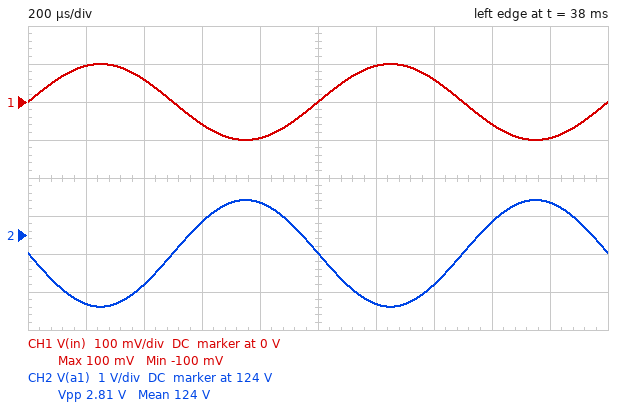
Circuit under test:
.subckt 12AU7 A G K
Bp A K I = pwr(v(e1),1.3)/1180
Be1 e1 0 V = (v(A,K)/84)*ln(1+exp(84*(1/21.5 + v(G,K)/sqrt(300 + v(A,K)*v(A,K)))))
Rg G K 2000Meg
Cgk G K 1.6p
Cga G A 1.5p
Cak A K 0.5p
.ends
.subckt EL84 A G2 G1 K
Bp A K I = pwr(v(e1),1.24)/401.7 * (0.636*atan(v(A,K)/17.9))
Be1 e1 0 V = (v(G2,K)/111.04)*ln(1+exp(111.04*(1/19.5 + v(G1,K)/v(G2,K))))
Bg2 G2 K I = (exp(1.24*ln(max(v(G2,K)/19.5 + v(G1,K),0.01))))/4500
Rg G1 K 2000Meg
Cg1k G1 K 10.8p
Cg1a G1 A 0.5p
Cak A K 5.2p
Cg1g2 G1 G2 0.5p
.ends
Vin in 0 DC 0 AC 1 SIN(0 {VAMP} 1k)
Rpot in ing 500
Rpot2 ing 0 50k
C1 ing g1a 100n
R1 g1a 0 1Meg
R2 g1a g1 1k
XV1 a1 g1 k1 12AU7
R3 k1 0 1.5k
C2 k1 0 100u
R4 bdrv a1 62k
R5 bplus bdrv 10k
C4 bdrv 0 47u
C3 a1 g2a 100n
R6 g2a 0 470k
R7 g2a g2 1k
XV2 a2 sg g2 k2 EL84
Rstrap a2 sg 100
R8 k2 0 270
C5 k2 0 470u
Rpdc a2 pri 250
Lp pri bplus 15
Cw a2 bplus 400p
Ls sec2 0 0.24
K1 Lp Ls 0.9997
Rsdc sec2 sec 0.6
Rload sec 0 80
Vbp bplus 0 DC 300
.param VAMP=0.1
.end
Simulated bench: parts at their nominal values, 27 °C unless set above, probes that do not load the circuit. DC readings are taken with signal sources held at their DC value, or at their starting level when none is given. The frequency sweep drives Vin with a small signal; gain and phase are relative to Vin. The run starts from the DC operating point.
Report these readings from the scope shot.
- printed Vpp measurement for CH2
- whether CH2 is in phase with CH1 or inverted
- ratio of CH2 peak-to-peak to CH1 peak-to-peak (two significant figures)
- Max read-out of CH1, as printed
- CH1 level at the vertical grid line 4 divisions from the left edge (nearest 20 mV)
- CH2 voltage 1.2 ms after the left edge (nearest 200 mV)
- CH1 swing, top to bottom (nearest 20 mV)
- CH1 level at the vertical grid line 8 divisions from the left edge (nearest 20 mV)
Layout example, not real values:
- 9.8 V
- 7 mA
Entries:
- 2.81 V
- inverted
- 14
- 100 mV
- -100 mV
- 122.2 V
- 200 mV
- -60 mV
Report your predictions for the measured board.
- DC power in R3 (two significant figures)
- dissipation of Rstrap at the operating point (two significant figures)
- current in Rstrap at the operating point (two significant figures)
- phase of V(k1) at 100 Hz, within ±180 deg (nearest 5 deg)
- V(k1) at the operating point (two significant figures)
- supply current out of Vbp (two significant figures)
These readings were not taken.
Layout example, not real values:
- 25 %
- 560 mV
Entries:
- 9.0 mW
- 570 µW
- 2.4 mA
- -90 deg
- 3.7 V
- 31 mA
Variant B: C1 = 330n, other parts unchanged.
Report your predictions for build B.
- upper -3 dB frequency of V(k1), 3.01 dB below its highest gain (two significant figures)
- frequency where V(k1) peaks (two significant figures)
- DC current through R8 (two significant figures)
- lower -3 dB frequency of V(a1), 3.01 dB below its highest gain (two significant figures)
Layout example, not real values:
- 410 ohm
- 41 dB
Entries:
- 2.4 Hz
- 870 mHz
- 29 mA
- 810 mHz
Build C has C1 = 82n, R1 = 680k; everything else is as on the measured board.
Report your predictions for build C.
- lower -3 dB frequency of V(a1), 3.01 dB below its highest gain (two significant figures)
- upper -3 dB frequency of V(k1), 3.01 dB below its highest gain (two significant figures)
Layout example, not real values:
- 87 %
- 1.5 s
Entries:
- 3.1 Hz
- 5.5 Hz
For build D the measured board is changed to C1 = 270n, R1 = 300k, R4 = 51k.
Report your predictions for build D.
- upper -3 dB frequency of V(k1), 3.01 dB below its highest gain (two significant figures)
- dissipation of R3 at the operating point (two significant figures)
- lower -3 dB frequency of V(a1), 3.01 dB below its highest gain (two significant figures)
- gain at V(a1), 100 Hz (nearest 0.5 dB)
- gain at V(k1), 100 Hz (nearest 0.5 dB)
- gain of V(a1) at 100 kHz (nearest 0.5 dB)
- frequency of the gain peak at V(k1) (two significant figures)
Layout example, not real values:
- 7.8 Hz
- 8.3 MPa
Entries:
- 4.4 Hz
- 11 mW
- 2.3 Hz
- 22.5 dB
- -46.5 dB
- 22.0 dB
- 1.8 Hz
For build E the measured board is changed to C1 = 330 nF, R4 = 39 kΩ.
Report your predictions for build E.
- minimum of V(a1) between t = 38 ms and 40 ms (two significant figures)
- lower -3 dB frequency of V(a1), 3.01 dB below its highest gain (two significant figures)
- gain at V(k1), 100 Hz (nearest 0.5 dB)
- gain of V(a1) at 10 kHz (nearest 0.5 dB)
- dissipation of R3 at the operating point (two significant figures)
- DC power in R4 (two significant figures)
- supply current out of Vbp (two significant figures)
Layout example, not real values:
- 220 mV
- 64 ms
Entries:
- 150 V
- 1.0 Hz
- -45.0 dB
- 22.0 dB
- 14 mW
- 360 mW
- 32 mA
